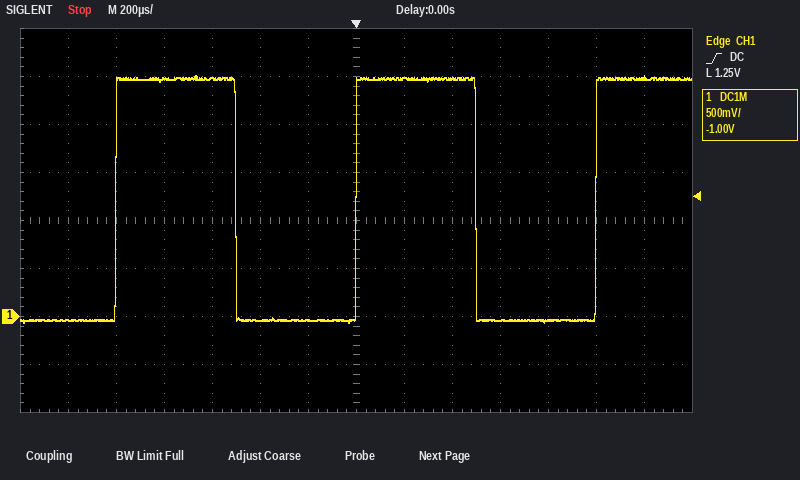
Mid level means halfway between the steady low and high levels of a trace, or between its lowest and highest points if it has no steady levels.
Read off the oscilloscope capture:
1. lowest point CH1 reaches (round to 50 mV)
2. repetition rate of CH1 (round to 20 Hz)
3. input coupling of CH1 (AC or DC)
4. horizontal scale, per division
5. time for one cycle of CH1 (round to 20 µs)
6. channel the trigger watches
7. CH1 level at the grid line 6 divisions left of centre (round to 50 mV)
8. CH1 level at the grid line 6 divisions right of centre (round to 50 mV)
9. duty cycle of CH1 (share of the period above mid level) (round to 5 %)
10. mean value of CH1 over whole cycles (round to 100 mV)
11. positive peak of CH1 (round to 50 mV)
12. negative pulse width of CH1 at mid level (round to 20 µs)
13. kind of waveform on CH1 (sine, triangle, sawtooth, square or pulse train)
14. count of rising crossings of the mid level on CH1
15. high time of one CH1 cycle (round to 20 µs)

-50 mV
1.00 kHz
DC
200 µs
1.00 ms
CH1
-50 mV
2.50 V
50 %
1.2 V
2.50 V
500 µs
square
3
500 µs
